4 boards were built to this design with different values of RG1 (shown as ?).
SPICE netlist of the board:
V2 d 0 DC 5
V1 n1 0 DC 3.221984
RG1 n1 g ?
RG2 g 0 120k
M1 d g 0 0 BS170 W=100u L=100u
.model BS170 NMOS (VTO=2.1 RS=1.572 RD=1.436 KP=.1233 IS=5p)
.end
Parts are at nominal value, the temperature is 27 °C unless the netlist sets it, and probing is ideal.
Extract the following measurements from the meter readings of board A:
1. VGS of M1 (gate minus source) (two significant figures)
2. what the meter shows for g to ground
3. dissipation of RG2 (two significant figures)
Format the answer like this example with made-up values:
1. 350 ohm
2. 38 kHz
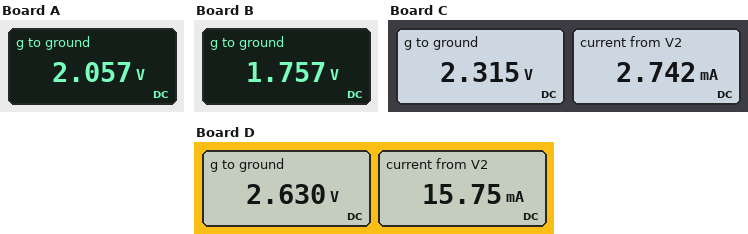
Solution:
1. 2.1 V
2. 2.057 V
3. 35 µW
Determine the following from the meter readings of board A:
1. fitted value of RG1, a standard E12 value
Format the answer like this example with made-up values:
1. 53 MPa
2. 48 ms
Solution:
1. 68 kΩ
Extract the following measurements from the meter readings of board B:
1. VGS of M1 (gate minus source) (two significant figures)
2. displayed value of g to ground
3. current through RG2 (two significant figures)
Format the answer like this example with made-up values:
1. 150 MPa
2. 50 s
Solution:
1. 1.8 V
2. 1.757 V
3. 15 µA
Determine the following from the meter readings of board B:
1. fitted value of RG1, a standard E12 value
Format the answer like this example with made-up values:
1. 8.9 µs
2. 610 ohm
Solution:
1. 100 kΩ
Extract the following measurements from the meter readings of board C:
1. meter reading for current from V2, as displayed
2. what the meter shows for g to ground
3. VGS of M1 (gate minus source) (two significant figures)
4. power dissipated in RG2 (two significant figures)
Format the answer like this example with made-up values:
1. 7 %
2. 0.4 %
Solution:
1. 2.742 mA
2. 2.315 V
3. 2.3 V
4. 45 µW
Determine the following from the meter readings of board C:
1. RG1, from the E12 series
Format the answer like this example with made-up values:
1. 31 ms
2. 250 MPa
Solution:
1. 47 kΩ
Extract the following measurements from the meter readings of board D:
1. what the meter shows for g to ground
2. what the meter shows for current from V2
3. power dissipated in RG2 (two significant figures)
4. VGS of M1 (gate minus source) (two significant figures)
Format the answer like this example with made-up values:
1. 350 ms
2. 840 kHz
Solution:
1. 2.630 V
2. 15.75 mA
3. 58 µW
4. 2.6 V
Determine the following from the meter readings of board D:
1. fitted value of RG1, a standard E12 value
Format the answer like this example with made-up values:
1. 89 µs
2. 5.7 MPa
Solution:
1. 27 kΩ
